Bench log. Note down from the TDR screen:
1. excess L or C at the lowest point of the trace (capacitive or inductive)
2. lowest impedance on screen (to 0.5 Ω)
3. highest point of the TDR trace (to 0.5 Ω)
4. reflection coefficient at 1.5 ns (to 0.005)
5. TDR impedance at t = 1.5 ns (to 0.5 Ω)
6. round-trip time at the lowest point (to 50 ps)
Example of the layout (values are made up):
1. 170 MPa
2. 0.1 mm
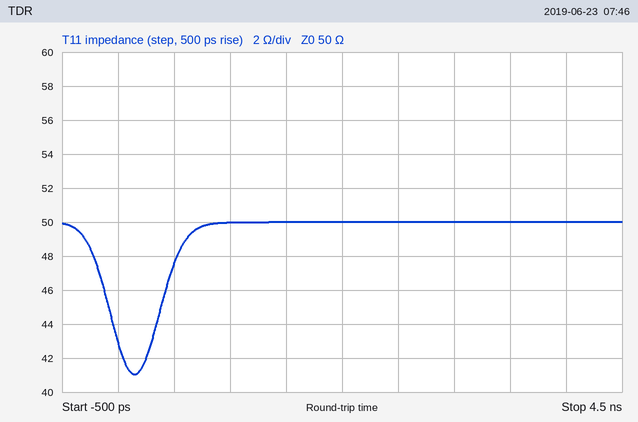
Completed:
1. capacitive
2. 41.0 Ω
3. 50.0 Ω
4. 0.000
5. 50.0 Ω
6. 150 ps
